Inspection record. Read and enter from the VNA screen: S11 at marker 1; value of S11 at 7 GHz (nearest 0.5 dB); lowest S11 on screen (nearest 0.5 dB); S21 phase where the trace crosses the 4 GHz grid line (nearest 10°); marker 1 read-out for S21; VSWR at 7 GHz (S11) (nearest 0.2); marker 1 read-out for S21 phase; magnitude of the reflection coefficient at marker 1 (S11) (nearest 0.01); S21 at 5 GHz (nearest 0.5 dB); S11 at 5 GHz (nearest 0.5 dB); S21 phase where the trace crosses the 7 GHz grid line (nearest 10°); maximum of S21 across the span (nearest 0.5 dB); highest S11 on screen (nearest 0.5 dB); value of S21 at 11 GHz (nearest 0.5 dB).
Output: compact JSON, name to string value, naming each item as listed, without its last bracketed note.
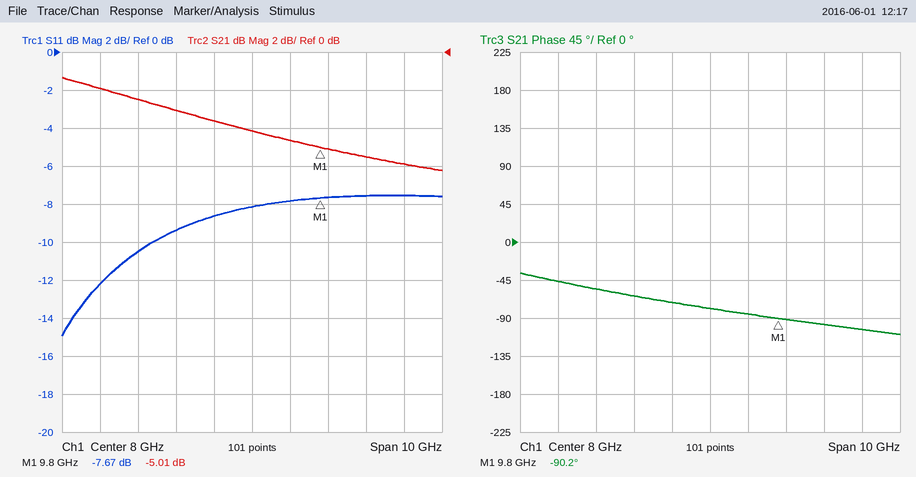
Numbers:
{"S11 at marker 1": "-7.67 dB", "value of S11 at 7 GHz": "-8.5 dB", "lowest S11 on screen": "-15.0 dB", "S21 phase where the trace crosses the 4 GHz grid line": "-50°", "marker 1 read-out for S21": "-5.01 dB", "VSWR at 7 GHz (S11)": "2.2", "marker 1 read-out for S21 phase": "-90.2°", "magnitude of the reflection coefficient at marker 1 (S11)": "0.41", "S21 at 5 GHz": "-2.5 dB", "S11 at 5 GHz": "-10.5 dB", "S21 phase where the trace crosses the 7 GHz grid line": "-70°", "maximum of S21 across the span": "-1.5 dB", "highest S11 on screen": "-7.5 dB", "value of S21 at 11 GHz": "-5.5 dB"}
